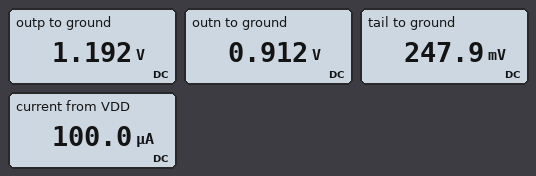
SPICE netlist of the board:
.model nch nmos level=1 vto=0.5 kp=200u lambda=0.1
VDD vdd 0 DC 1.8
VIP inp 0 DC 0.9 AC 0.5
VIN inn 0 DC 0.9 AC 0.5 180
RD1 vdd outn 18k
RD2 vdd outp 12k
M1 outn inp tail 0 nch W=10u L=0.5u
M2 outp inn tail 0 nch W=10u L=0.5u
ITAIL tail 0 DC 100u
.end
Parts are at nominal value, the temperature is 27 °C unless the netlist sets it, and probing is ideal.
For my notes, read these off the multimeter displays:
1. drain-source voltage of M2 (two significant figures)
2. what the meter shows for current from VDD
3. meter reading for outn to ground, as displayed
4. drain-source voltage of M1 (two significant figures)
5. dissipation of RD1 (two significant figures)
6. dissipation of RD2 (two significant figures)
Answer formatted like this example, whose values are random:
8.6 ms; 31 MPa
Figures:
940 mV; 100.0 µA; 0.912 V; 660 mV; 44 µW; 31 µW
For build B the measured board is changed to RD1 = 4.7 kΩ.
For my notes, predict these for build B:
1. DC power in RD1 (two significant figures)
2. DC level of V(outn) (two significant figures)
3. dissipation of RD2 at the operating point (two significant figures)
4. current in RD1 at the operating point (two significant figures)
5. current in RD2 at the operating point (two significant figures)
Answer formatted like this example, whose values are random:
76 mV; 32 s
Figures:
12 µW; 1.6 V; 29 µW; 51 µA; 49 µA
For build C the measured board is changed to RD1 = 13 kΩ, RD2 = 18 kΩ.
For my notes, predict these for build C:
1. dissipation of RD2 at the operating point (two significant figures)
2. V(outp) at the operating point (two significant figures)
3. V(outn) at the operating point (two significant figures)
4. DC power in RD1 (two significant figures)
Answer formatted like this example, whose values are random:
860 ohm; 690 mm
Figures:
44 µW; 910 mV; 1.1 V; 33 µW
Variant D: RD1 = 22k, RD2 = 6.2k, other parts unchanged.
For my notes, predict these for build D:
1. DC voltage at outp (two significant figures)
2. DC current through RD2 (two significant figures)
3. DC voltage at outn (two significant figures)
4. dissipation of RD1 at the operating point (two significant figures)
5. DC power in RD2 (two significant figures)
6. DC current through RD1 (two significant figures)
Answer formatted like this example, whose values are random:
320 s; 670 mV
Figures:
1.5 V; 52 µA; 740 mV; 51 µW; 17 µW; 48 µA
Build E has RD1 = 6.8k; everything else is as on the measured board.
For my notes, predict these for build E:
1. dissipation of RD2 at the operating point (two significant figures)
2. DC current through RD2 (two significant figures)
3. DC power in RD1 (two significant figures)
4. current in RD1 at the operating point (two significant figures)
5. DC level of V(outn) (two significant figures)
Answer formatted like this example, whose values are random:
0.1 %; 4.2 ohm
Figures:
29 µW; 49 µA; 17 µW; 51 µA; 1.5 V
